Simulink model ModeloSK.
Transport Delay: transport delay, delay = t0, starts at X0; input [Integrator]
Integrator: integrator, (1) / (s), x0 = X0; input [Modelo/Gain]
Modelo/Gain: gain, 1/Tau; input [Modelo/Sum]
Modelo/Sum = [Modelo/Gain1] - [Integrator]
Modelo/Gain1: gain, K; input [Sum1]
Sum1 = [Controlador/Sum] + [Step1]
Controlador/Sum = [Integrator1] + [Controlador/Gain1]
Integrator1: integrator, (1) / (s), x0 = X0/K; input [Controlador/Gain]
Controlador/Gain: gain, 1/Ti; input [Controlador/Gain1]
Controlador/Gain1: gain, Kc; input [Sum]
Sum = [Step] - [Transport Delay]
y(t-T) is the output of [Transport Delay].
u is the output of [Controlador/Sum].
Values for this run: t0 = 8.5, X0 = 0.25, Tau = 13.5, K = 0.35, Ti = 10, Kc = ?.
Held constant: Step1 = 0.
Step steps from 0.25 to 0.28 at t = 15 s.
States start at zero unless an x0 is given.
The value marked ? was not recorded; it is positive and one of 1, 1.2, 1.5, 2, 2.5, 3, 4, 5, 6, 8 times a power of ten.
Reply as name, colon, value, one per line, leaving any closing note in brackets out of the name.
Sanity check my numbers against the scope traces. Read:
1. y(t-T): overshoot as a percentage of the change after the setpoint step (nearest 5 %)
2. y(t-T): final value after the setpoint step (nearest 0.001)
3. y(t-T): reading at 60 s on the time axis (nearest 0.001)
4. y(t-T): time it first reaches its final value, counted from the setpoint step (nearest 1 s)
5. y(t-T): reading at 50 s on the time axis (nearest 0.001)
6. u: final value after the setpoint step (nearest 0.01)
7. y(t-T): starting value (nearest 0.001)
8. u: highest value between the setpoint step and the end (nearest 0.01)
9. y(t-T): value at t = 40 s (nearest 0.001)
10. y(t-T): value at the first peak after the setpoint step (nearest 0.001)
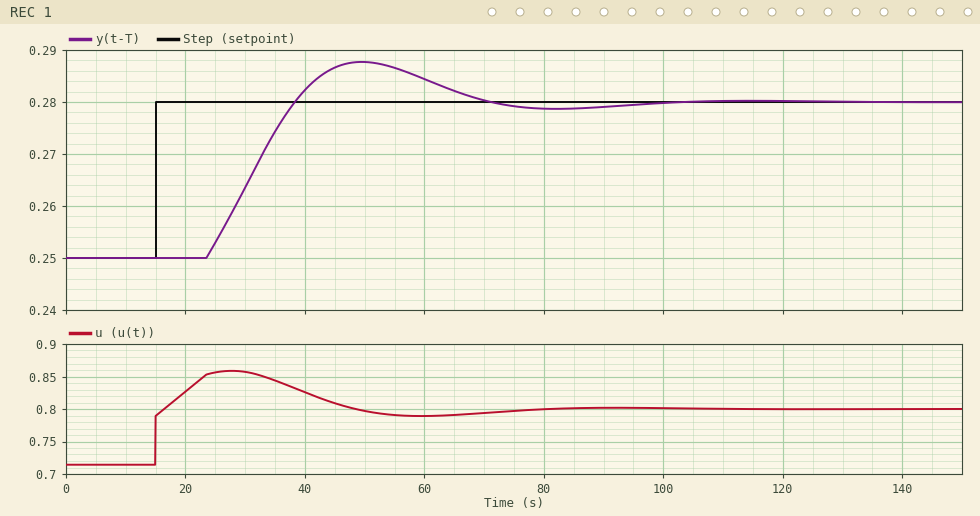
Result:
y(t-T): overshoot as a percentage of the change after the setpoint step: 25 %
y(t-T): final value after the setpoint step: 0.280
y(t-T): reading at 60 s on the time axis: 0.284
y(t-T): time it first reaches its final value, counted from the setpoint step: 23 s
y(t-T): reading at 50 s on the time axis: 0.288
u: final value after the setpoint step: 0.80
y(t-T): starting value: 0.250
u: highest value between the setpoint step and the end: 0.86
y(t-T): value at t = 40 s: 0.282
y(t-T): value at the first peak after the setpoint step: 0.288
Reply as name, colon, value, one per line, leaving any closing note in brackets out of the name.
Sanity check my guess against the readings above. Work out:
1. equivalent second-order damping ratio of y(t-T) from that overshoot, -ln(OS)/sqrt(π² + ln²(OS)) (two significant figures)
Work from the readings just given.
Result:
equivalent second-order damping ratio of y(t-T) from that overshoot, -ln(OS)/sqrt(π² + ln²(OS)): 0.40
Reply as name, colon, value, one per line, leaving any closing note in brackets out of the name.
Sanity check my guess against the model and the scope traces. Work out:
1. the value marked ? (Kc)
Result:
the value marked ?: 2.5
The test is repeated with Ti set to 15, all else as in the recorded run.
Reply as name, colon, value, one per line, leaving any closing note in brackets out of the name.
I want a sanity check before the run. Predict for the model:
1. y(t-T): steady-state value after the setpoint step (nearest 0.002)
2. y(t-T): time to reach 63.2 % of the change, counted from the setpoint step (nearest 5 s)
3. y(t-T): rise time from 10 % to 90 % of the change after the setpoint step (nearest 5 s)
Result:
y(t-T): steady-state value after the setpoint step: 0.280
y(t-T): time to reach 63.2 % of the change, counted from the setpoint step: 20 s
y(t-T): rise time from 10 % to 90 % of the change after the setpoint step: 15 s
